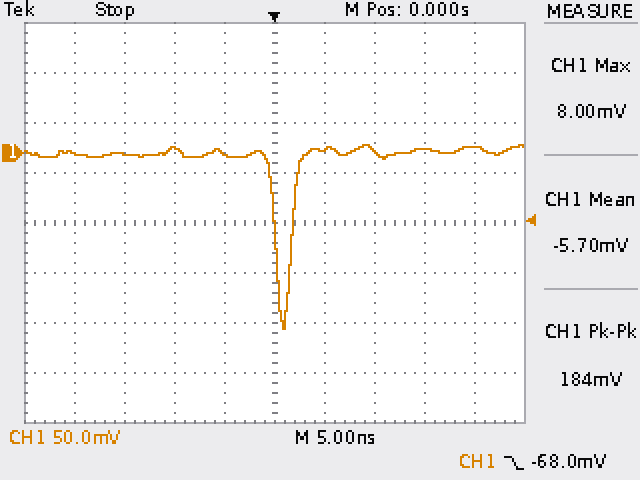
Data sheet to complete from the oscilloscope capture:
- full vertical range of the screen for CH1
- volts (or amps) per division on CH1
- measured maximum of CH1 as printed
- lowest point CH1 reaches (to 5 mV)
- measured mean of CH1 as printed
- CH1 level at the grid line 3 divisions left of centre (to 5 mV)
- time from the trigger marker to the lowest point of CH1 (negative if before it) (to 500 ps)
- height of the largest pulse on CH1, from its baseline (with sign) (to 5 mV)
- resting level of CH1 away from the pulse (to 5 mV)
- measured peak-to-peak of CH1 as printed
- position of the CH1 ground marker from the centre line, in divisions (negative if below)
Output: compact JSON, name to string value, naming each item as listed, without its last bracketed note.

{"full vertical range of the screen for CH1": "400 mV", "volts (or amps) per division on CH1": "50 mV", "measured maximum of CH1 as printed": "8.00 mV", "lowest point CH1 reaches": "-175 mV", "measured mean of CH1 as printed": "-5.70 mV", "CH1 level at the grid line 3 divisions left of centre": "0 mV", "time from the trigger marker to the lowest point of CH1 (negative if before it)": "+1.0 ns", "height of the largest pulse on CH1, from its baseline (with sign)": "-175 mV", "resting level of CH1 away from the pulse": "0 mV", "measured peak-to-peak of CH1 as printed": "184 mV", "position of the CH1 ground marker from the centre line, in divisions": "+1.4 div"}
